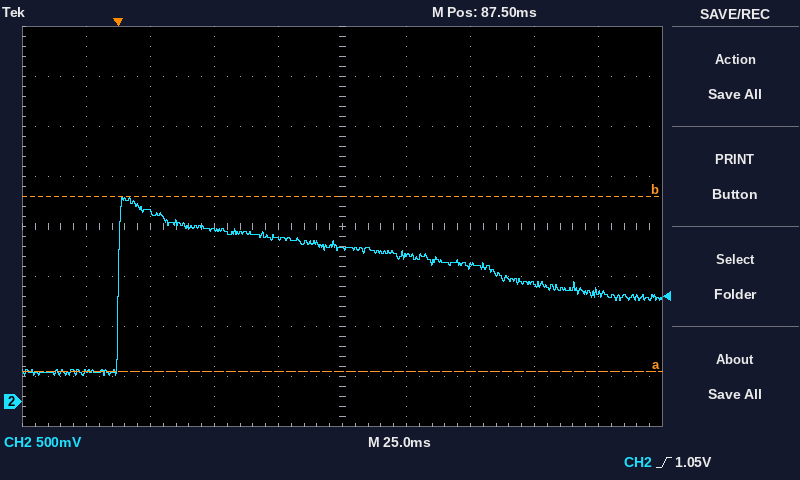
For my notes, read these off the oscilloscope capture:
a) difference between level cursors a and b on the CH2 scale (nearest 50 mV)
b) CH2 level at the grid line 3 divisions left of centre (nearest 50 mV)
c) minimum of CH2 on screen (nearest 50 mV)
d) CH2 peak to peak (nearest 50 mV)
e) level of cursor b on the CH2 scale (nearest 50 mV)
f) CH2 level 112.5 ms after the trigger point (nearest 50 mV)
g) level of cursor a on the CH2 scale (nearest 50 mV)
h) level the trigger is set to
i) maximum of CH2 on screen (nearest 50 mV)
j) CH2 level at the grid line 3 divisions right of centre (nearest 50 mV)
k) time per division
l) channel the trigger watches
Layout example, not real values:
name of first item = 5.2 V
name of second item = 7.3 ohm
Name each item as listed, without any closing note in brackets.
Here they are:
difference between level cursors a and b on the CH2 scale = 1.75 V
CH2 level at the grid line 3 divisions left of centre = 1.90 V
minimum of CH2 on screen = 250 mV
CH2 peak to peak = 1.80 V
level of cursor b on the CH2 scale = 2.05 V
CH2 level 112.5 ms after the trigger point = 1.45 V
level of cursor a on the CH2 scale = 300 mV
level the trigger is set to = 1.05 V
maximum of CH2 on screen = 2.05 V
CH2 level at the grid line 3 divisions right of centre = 1.15 V
time per division = 25 ms
channel the trigger watches = CH2
